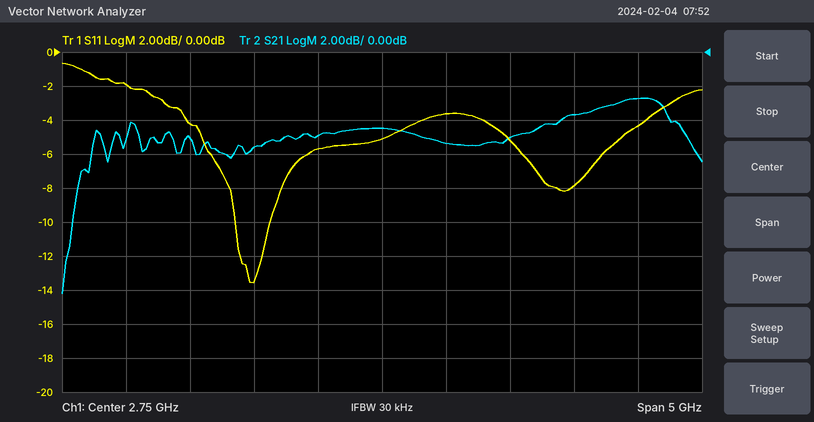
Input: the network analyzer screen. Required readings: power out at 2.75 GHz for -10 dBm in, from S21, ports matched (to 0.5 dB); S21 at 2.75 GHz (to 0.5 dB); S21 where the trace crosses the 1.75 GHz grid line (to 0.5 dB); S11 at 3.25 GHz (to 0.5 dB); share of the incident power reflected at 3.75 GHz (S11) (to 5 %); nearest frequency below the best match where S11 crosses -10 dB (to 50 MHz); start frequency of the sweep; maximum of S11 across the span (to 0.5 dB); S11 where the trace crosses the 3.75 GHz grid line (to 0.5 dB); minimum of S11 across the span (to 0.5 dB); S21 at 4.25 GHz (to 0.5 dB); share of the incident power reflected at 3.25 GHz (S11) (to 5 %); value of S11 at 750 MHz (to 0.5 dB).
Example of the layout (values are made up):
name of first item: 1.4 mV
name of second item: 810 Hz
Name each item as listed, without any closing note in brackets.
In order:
power out at 2.75 GHz for -10 dBm in, from S21, ports matched: -14.5 dBm
S21 at 2.75 GHz: -4.5 dB
S21 where the trace crosses the 1.75 GHz grid line: -5.5 dB
S11 at 3.25 GHz: -3.5 dB
share of the incident power reflected at 3.75 GHz (S11): 30 %
nearest frequency below the best match where S11 crosses -10 dB: 1.60 GHz
start frequency of the sweep: 250 MHz
maximum of S11 across the span: -0.5 dB
S11 where the trace crosses the 3.75 GHz grid line: -5.0 dB
minimum of S11 across the span: -13.5 dB
S21 at 4.25 GHz: -3.5 dB
share of the incident power reflected at 3.25 GHz (S11): 45 %
value of S11 at 750 MHz: -2.0 dB
